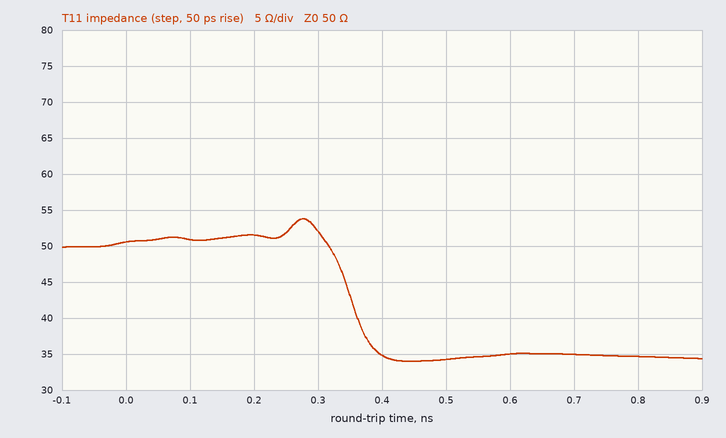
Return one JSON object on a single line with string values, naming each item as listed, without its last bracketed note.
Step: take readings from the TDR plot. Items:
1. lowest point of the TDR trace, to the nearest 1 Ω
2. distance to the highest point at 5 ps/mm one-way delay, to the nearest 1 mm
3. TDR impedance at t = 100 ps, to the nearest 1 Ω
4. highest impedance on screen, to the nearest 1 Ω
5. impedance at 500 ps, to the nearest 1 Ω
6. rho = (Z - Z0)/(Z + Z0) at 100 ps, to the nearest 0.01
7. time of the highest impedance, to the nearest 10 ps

{"lowest point of the TDR trace, to the nearest 1 Ω": "34 Ω", "distance to the highest point at 5 ps/mm one-way delay, to the nearest 1 mm": "28 mm", "TDR impedance at t = 100 ps, to the nearest 1 Ω": "51 Ω", "highest impedance on screen, to the nearest 1 Ω": "54 Ω", "impedance at 500 ps, to the nearest 1 Ω": "34 Ω", "rho = (Z - Z0)/(Z + Z0) at 100 ps, to the nearest 0.01": "+0.01", "time of the highest impedance, to the nearest 10 ps": "280 ps"}
